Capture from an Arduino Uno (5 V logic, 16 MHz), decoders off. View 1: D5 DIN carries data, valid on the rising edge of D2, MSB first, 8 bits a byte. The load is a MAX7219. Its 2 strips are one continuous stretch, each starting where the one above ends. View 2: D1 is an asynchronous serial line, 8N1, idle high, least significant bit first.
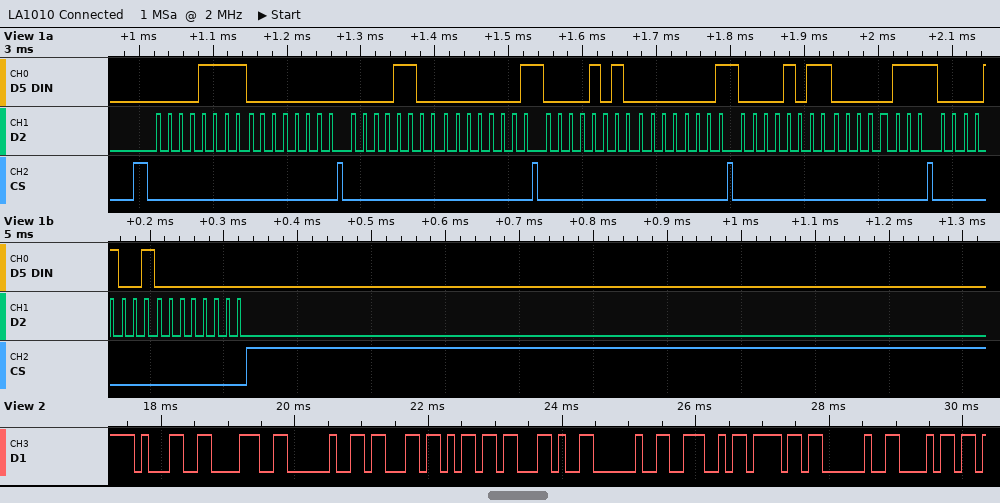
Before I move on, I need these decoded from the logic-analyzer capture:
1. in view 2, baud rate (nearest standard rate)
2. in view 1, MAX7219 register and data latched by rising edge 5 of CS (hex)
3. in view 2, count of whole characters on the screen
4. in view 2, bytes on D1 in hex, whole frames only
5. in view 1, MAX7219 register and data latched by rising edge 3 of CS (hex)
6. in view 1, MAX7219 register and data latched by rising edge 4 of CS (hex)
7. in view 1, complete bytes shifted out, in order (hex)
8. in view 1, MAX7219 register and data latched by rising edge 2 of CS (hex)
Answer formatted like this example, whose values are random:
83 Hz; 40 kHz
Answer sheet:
9600 baud; register 0xB, data 0x07; 11; 31 38 20 63 6D 2C 20 4E 6F 20 68; register 0xC, data 0x01; register 0xA, data 0x01; 0F 00 0C 01 0A 01 0B 07 09 00; register 0xF, data 0x00
